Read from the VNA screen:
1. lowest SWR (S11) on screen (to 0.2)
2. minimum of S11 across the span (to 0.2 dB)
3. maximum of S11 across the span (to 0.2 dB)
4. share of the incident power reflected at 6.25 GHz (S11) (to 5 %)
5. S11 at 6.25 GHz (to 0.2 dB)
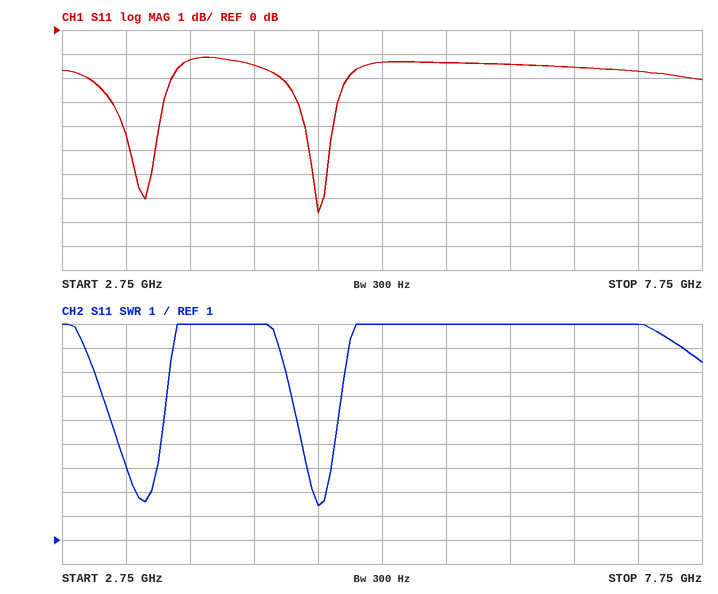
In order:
2.4
-7.6 dB
-1.2 dB
70 %
-1.4 dB
